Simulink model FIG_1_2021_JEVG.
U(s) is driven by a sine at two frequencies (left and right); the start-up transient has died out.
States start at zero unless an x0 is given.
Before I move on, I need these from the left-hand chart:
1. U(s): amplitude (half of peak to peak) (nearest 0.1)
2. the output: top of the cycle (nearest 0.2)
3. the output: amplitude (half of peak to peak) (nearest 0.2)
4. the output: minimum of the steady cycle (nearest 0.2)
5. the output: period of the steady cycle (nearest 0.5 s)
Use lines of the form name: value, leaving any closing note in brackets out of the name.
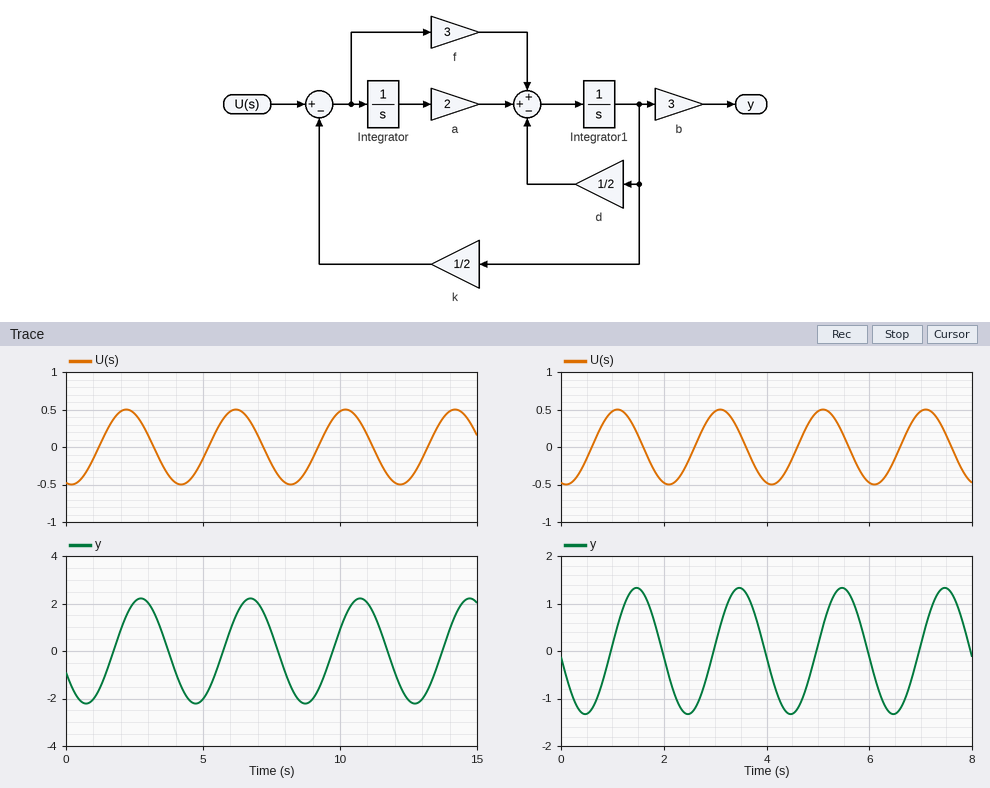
U(s): amplitude (half of peak to peak): 0.5
the output: top of the cycle: 2.2
the output: amplitude (half of peak to peak): 2.2
the output: minimum of the steady cycle: -2.2
the output: period of the steady cycle: 4.0 s
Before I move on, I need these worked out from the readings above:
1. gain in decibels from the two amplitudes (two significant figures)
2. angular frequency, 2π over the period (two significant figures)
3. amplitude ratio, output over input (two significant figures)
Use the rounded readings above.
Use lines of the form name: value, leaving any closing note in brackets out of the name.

gain in decibels from the two amplitudes: 13 dB
angular frequency, 2π over the period: 1.6 rad/s
amplitude ratio, output over input: 4.4
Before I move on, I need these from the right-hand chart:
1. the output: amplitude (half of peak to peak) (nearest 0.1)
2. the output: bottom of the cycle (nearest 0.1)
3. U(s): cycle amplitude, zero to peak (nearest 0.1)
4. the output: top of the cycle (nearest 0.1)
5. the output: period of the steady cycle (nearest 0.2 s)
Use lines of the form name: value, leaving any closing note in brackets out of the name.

the output: amplitude (half of peak to peak): 1.3
the output: bottom of the cycle: -1.3
U(s): cycle amplitude, zero to peak: 0.5
the output: top of the cycle: 1.3
the output: period of the steady cycle: 2.0 s
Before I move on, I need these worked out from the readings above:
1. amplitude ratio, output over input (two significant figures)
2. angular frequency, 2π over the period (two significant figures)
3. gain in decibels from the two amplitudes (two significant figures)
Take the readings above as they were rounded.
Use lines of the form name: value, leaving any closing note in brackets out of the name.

amplitude ratio, output over input: 2.6
angular frequency, 2π over the period: 3.1 rad/s
gain in decibels from the two amplitudes: 8.3 dB
